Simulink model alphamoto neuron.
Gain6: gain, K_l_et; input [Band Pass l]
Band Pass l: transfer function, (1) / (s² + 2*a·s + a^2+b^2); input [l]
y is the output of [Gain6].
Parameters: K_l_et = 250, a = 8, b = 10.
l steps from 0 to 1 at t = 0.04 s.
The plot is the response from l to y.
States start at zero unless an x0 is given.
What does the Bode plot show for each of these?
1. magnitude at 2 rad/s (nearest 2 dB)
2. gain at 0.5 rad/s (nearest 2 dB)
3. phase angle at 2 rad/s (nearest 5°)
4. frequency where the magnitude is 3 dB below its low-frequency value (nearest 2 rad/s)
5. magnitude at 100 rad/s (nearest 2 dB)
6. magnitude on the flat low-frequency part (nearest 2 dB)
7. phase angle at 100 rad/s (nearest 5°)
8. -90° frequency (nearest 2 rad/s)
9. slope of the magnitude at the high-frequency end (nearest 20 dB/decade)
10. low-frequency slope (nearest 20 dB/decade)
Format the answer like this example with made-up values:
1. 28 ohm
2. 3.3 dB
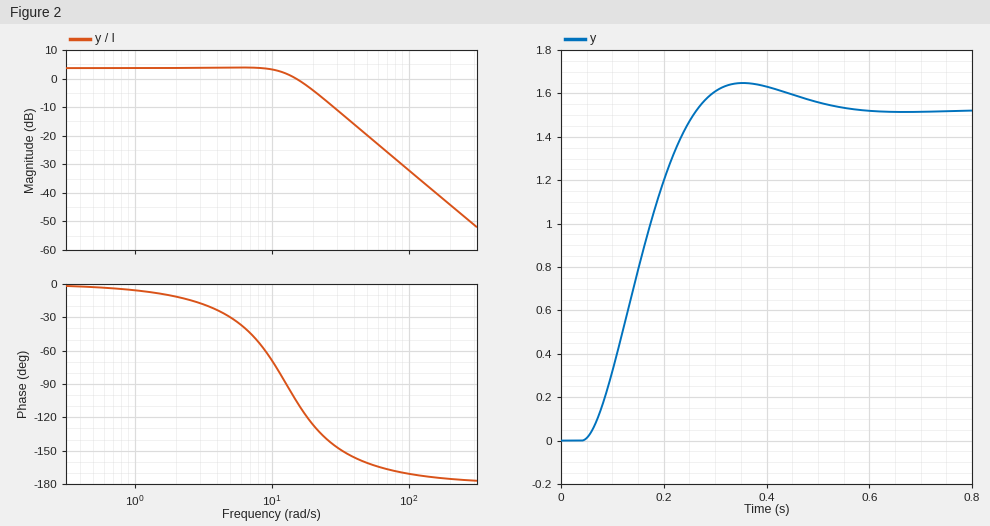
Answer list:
1. 4 dB
2. 4 dB
3. -10°
4. 14 rad/s
5. -32 dB
6. 4 dB
7. -170°
8. 12 rad/s
9. -40 dB/decade
10. 0 dB/decade
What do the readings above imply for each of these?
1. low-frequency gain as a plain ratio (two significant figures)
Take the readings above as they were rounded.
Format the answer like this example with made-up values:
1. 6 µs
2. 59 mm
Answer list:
1. 1.6
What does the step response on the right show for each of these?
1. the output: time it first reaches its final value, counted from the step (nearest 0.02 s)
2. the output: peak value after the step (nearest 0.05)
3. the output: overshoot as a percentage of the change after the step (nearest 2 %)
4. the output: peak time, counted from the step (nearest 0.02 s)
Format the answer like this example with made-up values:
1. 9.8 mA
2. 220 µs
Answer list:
1. 0.22 s
2. 1.65
3. 8 %
4. 0.32 s
